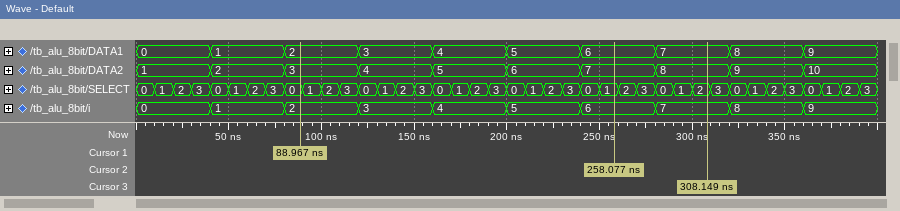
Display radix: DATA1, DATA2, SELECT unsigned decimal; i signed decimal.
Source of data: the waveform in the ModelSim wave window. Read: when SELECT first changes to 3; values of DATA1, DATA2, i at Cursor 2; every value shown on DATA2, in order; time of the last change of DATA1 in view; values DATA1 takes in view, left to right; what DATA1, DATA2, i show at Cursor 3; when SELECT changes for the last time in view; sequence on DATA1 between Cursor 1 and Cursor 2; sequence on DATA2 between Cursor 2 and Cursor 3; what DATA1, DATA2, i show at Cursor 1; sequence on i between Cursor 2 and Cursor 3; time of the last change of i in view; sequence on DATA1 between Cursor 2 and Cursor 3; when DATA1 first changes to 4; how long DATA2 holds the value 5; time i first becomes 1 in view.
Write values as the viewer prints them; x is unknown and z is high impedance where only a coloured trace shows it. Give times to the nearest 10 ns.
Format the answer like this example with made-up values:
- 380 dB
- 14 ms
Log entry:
- 30 ns
- DATA1=6, DATA2=7, i=6
- 1, 2, 3, 4, 5, 6, 7, 8, 9, 10
- 360 ns
- 0, 1, 2, 3, 4, 5, 6, 7, 8, 9
- DATA1=7, DATA2=8, i=7
- 390 ns
- 2, 3, 4, 5, 6
- 7, 8
- DATA1=2, DATA2=3, i=2
- 6, 7
- 360 ns
- 6, 7
- 160 ns
- 40 ns
- 40 ns
